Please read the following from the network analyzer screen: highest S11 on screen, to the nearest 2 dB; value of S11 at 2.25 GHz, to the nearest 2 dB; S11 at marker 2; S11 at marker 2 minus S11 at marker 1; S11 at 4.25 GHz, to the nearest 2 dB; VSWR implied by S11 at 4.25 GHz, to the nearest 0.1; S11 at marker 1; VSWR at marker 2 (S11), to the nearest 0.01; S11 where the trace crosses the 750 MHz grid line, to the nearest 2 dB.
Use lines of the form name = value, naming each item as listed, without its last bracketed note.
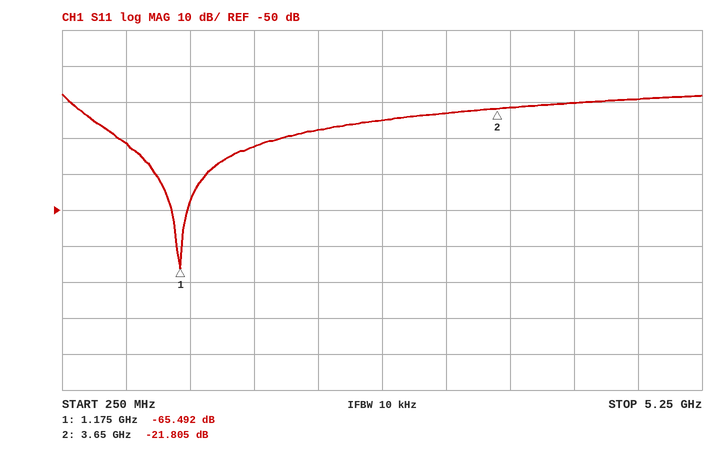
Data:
highest S11 on screen, to the nearest 2 dB = -18 dB
value of S11 at 2.25 GHz, to the nearest 2 dB = -28 dB
S11 at marker 2 = -21.805 dB
S11 at marker 2 minus S11 at marker 1 = 43.687 dB
S11 at 4.25 GHz, to the nearest 2 dB = -20 dB
VSWR implied by S11 at 4.25 GHz, to the nearest 0.1 = 1.2
S11 at marker 1 = -65.492 dB
VSWR at marker 2 (S11), to the nearest 0.01 = 1.18
S11 where the trace crosses the 750 MHz grid line, to the nearest 2 dB = -32 dB
